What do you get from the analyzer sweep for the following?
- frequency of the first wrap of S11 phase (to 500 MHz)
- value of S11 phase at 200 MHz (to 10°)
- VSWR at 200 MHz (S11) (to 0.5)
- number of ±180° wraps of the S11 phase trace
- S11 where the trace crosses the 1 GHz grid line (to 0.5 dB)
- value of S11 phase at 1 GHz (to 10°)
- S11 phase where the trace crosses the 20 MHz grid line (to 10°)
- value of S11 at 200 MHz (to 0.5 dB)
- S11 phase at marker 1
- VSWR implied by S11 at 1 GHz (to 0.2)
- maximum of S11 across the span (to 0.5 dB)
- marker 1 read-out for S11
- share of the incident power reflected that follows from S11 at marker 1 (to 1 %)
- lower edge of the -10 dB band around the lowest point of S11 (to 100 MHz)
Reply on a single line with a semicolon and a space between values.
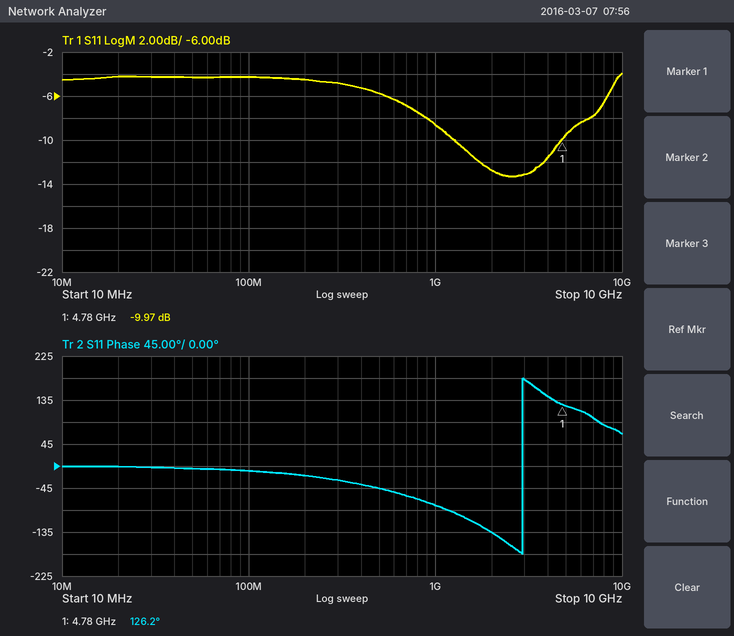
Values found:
3.0 GHz; -20°; 4.0; 1; -8.5 dB; -80°; 0°; -4.5 dB; 126.2°; 2.2; -4.0 dB; -9.97 dB; 10 %; 1.3 GHz
